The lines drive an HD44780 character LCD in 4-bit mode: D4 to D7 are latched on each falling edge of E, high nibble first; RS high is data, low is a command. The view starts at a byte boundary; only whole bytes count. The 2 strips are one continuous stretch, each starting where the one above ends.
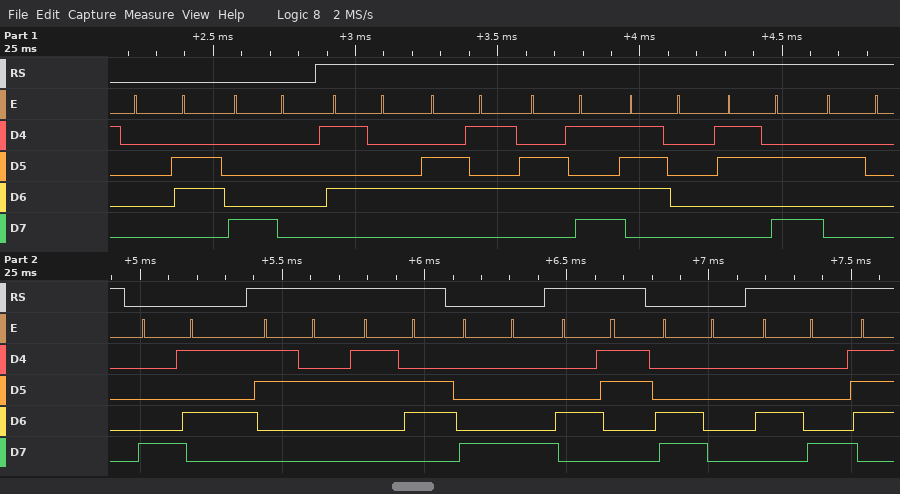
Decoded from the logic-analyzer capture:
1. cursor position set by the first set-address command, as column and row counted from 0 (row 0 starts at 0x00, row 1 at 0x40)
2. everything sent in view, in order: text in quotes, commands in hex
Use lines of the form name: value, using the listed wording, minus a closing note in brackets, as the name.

cursor position set by the first set-address command, as column and row counted from 0: column 0, row 0
everything sent in view, in order: text in quotes, commands in hex: 0x06 0x80 "Temp: " 0x85 "26" 0x88 "C" 0xC0 "H"
